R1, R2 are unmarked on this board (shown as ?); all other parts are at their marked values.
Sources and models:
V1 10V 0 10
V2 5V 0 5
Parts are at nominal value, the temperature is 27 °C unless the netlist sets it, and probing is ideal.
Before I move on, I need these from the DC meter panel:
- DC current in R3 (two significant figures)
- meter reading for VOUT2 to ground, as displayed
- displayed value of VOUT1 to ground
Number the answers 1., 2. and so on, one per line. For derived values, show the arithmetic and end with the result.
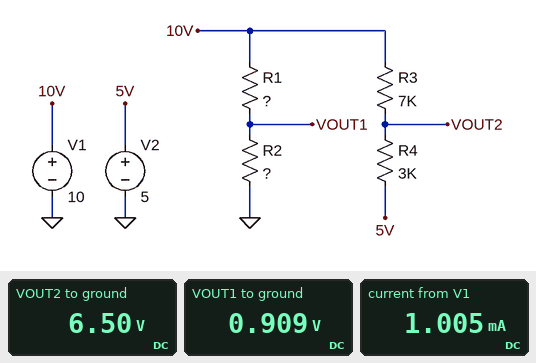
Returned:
1. (10 V - 6.5 V) / 7 kΩ = 500 µA
2. 6.50 V
3. 0.909 V
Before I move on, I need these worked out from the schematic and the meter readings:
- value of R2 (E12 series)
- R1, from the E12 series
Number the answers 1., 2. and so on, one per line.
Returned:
1. 1.8 kΩ
2. 18 kΩ
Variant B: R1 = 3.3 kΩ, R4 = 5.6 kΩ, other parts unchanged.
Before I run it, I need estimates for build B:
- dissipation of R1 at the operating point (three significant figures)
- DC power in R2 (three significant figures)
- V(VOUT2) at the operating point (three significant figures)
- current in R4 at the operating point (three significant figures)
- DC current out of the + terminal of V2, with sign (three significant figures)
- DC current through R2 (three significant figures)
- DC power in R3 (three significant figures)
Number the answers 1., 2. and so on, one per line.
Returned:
1. 12.7 mW
2. 6.92 mW
3. 7.22 V
4. 397 µA
5. -397 µA
6. 1.96 mA
7. 1.10 mW
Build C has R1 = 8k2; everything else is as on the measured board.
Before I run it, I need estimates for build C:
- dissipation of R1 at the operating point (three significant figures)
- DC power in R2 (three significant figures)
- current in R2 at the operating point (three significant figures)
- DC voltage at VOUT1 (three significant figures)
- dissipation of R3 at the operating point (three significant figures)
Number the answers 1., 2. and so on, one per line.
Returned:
1. 8.20 mW
2. 1.80 mW
3. 1.00 mA
4. 1.80 V
5. 1.75 mW
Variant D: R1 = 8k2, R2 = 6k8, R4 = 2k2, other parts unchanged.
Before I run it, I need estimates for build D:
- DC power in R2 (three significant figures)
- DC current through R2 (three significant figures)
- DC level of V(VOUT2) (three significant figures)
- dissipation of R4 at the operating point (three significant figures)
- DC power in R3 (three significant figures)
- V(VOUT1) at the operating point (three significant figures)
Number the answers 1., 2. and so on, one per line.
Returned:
1. 3.02 mW
2. 667 µA
3. 6.20 V
4. 650 µW
5. 2.07 mW
6. 4.53 V
